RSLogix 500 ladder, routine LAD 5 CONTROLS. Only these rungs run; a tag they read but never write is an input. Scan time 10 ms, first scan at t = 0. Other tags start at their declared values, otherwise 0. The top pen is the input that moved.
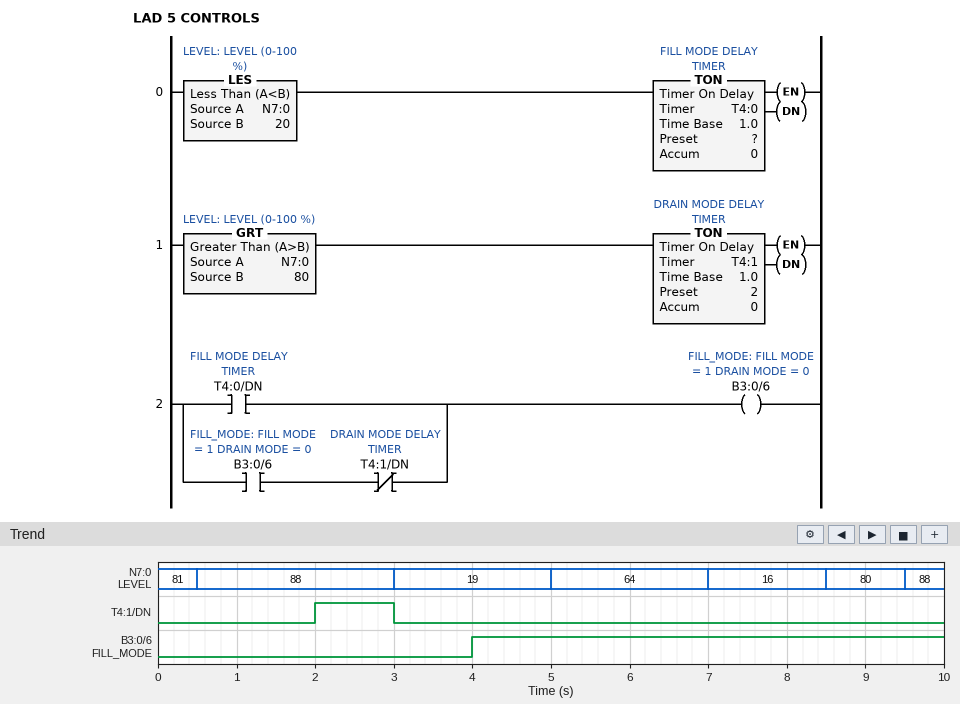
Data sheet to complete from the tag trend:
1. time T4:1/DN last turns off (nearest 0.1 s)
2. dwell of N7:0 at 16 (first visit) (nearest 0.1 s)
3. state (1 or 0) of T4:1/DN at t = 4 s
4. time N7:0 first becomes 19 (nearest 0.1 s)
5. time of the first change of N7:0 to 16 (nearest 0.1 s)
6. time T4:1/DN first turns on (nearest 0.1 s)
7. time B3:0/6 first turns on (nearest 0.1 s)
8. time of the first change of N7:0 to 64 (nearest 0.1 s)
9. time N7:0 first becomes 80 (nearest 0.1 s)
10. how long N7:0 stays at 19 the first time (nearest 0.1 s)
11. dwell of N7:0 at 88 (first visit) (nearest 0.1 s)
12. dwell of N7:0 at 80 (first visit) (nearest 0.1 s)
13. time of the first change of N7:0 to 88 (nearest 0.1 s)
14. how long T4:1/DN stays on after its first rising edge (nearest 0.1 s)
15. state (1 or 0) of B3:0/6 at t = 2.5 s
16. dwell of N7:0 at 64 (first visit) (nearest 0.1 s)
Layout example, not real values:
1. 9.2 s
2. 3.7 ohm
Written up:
1. 3.0 s
2. 1.5 s
3. 0
4. 3.0 s
5. 7.0 s
6. 2.0 s
7. 4.0 s
8. 5.0 s
9. 8.5 s
10. 2.0 s
11. 2.5 s
12. 1.0 s
13. 0.5 s
14. 1.0 s
15. 0
16. 2.0 s
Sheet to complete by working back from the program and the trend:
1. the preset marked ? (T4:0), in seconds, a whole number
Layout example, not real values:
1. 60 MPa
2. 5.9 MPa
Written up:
1. 1 s
